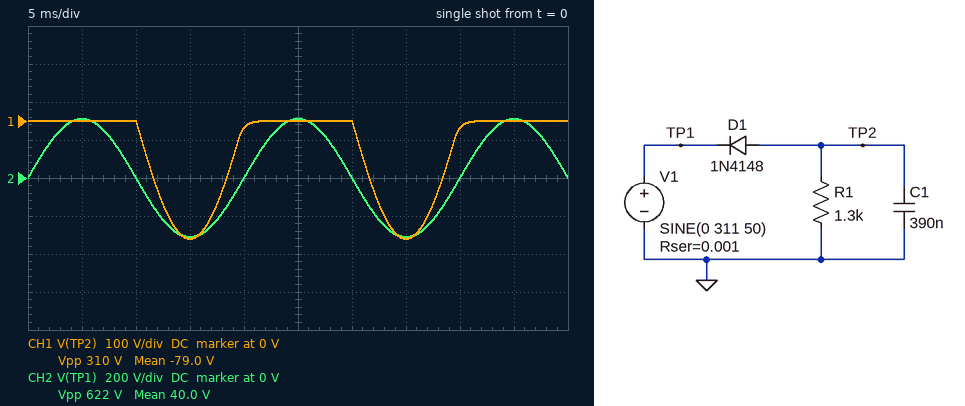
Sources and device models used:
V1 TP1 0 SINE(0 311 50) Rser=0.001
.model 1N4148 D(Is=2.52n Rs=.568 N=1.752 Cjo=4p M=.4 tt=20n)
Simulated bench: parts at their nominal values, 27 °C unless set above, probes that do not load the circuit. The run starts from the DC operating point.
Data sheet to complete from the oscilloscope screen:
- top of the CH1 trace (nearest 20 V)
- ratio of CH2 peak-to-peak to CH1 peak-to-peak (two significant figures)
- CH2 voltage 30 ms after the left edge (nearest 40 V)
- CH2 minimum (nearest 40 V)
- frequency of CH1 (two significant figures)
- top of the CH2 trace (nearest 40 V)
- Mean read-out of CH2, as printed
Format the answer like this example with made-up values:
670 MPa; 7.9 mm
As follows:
0 V; 2.0; 0 V; -320 V; 50 Hz; 320 V; 40.0 V
